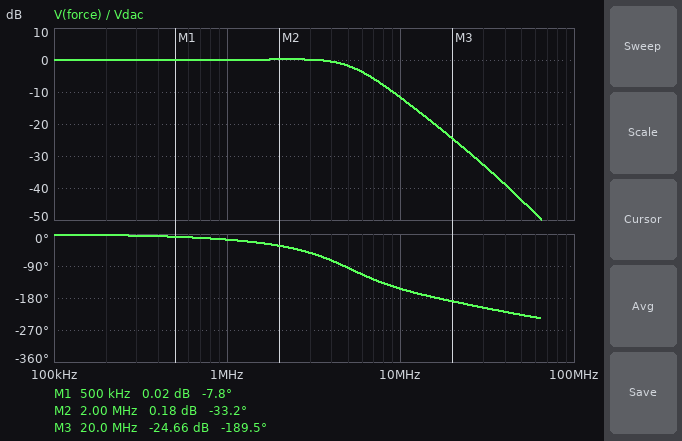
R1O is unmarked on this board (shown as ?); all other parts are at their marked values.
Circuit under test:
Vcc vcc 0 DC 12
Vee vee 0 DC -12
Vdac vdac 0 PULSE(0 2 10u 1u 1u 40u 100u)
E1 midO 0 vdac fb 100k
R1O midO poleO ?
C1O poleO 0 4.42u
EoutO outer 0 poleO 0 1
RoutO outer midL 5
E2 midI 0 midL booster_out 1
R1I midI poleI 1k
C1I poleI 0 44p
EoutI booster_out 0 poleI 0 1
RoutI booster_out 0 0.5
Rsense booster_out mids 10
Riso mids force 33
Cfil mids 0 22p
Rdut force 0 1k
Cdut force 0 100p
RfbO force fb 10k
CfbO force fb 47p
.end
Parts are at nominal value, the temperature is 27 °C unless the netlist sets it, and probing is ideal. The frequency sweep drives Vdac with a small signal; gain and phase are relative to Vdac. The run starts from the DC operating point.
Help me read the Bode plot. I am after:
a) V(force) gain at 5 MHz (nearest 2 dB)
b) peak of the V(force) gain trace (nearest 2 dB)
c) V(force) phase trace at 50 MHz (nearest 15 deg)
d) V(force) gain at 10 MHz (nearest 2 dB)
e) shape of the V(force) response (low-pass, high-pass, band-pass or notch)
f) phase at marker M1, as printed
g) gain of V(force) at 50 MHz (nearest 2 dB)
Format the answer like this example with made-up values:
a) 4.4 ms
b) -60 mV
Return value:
a) -2 dB
b) 0 dB
c) -225 deg
d) -12 dB
e) low-pass
f) -7.8 deg
g) -44 dB
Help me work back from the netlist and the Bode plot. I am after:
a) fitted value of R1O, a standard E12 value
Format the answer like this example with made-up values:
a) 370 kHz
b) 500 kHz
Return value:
a) 470 Ω
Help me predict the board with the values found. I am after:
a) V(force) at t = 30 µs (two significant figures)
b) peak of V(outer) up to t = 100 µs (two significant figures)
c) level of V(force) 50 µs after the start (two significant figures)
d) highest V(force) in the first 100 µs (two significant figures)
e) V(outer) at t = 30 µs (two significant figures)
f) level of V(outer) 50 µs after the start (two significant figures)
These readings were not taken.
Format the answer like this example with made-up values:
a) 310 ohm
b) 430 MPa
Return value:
a) 2.0 V
b) 4.2 V
c) 2.0 V
d) 2.0 V
e) 4.2 V
f) 4.2 V
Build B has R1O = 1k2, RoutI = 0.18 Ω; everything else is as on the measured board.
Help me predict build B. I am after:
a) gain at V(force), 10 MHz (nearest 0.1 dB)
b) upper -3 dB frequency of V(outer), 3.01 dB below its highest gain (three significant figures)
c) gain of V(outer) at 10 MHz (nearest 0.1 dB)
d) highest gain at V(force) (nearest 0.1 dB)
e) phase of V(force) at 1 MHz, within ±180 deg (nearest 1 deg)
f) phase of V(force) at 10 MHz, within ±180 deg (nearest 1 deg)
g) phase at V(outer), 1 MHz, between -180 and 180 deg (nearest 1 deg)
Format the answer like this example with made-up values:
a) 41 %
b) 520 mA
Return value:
a) -21.1 dB
b) 1.99 MHz
c) -9.8 dB
d) 0 dB
e) -38 deg
f) -158 deg
g) -29 deg
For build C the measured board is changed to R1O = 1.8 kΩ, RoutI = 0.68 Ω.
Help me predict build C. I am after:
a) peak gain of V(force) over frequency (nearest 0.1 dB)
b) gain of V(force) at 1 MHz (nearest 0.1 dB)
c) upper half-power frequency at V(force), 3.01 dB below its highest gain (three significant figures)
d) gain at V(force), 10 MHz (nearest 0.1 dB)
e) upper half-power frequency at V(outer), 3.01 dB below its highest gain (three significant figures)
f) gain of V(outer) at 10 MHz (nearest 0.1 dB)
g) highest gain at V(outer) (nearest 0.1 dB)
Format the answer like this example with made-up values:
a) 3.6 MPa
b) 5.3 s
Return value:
a) 0 dB
b) -2.5 dB
c) 1.14 MHz
d) -24.8 dB
e) 1.17 MHz
f) -13.5 dB
g) 6.4 dB
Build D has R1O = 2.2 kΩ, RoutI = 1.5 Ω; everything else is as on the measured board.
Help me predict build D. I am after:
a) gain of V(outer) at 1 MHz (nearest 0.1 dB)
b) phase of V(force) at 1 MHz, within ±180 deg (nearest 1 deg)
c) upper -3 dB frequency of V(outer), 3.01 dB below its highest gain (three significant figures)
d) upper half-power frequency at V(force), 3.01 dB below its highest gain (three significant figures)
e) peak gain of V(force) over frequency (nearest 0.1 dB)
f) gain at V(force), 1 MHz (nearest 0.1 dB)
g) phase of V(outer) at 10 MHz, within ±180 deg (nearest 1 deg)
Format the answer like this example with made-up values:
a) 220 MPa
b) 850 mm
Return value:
a) 3.0 dB
b) -58 deg
c) 917 kHz
d) 902 kHz
e) 0 dB
f) -3.5 dB
g) -89 deg
